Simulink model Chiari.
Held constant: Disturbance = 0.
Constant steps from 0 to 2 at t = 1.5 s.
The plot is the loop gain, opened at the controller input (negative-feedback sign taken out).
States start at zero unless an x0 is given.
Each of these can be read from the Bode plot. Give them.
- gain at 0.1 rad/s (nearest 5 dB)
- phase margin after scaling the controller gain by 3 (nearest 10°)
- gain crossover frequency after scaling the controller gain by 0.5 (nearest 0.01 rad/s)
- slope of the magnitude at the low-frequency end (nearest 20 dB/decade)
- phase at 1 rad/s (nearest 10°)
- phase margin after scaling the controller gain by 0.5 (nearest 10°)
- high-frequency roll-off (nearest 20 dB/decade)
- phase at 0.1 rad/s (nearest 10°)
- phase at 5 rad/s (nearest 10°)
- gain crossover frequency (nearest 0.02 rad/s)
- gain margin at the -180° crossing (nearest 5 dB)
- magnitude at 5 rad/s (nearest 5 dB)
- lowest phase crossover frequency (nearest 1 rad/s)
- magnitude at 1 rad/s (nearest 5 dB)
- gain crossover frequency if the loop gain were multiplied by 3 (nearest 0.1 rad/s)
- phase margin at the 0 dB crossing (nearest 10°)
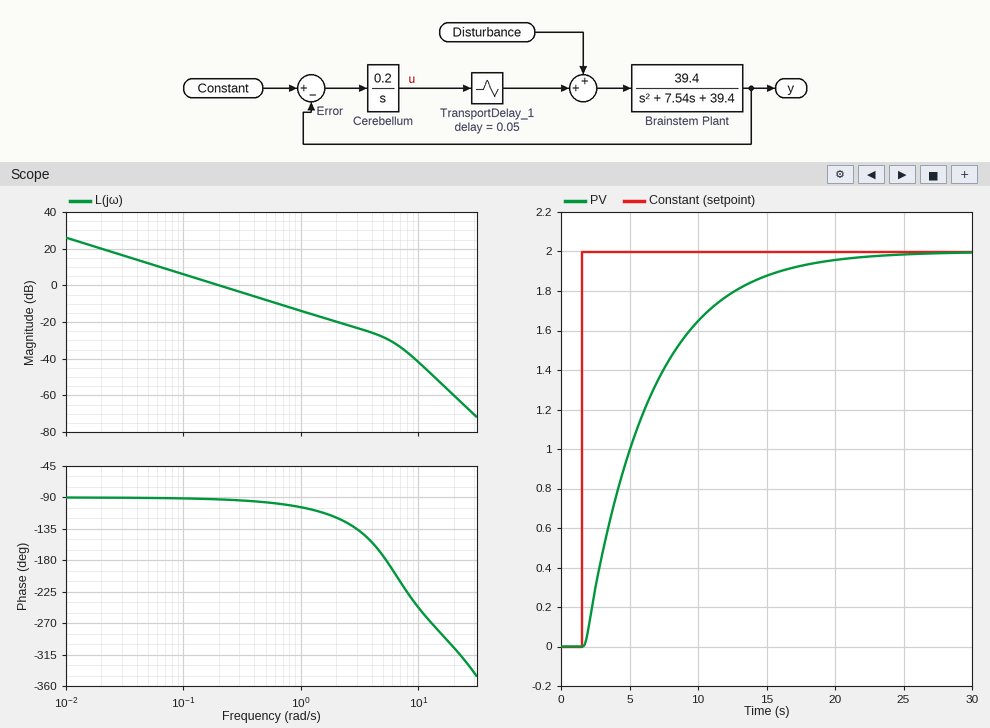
5 dB
80°
0.10 rad/s
-20 dB/decade
-100°
90°
-60 dB/decade
-90°
-170°
0.20 rad/s
30 dB
-30 dB
5 rad/s
-15 dB
0.6 rad/s
90°
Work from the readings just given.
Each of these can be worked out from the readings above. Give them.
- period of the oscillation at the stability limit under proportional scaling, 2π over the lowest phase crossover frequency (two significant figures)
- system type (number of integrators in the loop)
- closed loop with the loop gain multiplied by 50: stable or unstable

1.3 s
1
unstable
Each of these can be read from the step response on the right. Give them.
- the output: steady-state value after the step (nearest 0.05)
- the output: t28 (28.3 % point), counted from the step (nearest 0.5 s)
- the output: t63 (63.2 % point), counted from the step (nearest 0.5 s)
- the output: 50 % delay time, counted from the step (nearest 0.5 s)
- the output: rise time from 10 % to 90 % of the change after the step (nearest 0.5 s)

2.00
2.0 s
5.0 s
3.5 s
10.5 s
